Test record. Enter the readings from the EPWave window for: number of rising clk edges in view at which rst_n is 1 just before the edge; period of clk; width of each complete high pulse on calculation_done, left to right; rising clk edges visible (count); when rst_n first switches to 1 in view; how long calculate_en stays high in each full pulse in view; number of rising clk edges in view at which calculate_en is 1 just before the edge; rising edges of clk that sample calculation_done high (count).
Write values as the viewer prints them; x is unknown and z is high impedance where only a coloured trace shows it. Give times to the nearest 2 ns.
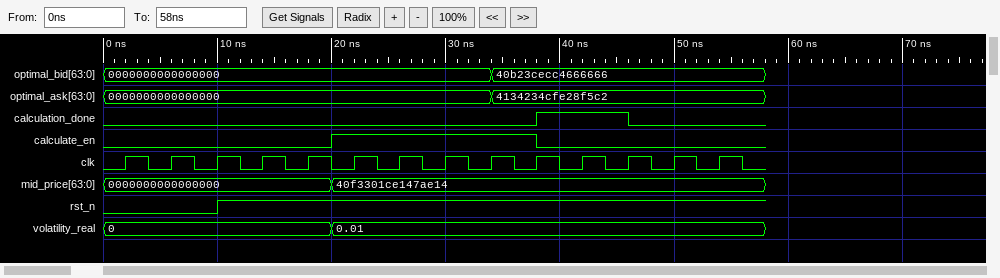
11
4 ns
8 ns
14
10 ns
18 ns
5
2
